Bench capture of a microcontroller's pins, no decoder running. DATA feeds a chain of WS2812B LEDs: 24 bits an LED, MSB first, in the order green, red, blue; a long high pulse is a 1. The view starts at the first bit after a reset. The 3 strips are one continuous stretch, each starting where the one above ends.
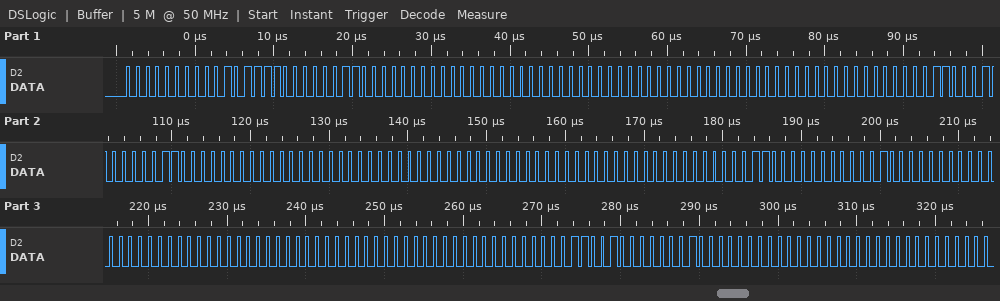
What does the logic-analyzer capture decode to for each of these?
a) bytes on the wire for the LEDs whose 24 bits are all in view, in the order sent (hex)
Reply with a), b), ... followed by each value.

a) 00 2F 03 00 00 00 00 00 00 00 31 03 00 00 00 00 00 00 00 30 01 00 00 00 00 00 00 00 32 02 00 00 00
